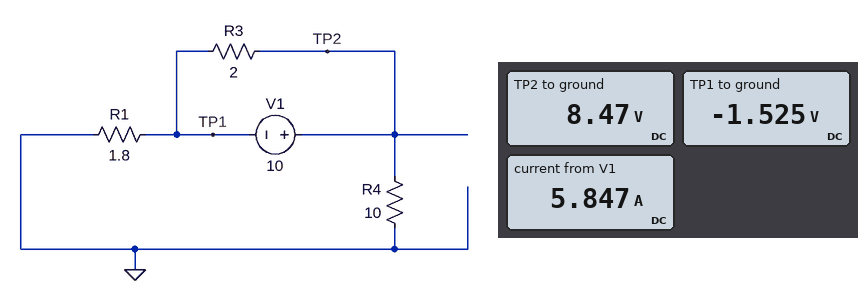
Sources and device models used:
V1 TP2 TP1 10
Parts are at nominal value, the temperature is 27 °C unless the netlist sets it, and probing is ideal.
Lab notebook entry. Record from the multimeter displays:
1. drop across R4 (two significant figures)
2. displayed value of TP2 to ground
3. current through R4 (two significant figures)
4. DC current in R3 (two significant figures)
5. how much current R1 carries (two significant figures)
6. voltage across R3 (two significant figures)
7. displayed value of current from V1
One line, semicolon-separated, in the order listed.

8.5 V; 8.47 V; 850 mA; 5.0 A; 850 mA; 10 V; 5.847 A
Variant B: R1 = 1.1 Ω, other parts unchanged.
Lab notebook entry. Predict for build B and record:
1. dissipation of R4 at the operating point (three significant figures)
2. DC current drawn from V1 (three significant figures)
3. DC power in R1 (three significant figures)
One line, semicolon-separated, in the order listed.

8.12 W; 5.90 A; 893 mW
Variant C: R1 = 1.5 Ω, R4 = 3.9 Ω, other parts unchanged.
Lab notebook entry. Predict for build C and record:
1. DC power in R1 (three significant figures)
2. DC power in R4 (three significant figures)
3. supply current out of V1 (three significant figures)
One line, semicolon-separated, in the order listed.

5.14 W; 13.4 W; 6.85 A
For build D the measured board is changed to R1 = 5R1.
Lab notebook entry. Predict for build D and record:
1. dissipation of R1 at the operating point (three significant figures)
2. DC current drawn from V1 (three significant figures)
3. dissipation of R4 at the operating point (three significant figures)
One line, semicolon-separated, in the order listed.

2.24 W; 5.66 A; 4.39 W
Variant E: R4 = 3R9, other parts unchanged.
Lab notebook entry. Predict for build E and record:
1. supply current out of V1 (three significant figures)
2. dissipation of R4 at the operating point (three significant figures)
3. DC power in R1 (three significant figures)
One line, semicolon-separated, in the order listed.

6.75 A; 12.0 W; 5.54 W
